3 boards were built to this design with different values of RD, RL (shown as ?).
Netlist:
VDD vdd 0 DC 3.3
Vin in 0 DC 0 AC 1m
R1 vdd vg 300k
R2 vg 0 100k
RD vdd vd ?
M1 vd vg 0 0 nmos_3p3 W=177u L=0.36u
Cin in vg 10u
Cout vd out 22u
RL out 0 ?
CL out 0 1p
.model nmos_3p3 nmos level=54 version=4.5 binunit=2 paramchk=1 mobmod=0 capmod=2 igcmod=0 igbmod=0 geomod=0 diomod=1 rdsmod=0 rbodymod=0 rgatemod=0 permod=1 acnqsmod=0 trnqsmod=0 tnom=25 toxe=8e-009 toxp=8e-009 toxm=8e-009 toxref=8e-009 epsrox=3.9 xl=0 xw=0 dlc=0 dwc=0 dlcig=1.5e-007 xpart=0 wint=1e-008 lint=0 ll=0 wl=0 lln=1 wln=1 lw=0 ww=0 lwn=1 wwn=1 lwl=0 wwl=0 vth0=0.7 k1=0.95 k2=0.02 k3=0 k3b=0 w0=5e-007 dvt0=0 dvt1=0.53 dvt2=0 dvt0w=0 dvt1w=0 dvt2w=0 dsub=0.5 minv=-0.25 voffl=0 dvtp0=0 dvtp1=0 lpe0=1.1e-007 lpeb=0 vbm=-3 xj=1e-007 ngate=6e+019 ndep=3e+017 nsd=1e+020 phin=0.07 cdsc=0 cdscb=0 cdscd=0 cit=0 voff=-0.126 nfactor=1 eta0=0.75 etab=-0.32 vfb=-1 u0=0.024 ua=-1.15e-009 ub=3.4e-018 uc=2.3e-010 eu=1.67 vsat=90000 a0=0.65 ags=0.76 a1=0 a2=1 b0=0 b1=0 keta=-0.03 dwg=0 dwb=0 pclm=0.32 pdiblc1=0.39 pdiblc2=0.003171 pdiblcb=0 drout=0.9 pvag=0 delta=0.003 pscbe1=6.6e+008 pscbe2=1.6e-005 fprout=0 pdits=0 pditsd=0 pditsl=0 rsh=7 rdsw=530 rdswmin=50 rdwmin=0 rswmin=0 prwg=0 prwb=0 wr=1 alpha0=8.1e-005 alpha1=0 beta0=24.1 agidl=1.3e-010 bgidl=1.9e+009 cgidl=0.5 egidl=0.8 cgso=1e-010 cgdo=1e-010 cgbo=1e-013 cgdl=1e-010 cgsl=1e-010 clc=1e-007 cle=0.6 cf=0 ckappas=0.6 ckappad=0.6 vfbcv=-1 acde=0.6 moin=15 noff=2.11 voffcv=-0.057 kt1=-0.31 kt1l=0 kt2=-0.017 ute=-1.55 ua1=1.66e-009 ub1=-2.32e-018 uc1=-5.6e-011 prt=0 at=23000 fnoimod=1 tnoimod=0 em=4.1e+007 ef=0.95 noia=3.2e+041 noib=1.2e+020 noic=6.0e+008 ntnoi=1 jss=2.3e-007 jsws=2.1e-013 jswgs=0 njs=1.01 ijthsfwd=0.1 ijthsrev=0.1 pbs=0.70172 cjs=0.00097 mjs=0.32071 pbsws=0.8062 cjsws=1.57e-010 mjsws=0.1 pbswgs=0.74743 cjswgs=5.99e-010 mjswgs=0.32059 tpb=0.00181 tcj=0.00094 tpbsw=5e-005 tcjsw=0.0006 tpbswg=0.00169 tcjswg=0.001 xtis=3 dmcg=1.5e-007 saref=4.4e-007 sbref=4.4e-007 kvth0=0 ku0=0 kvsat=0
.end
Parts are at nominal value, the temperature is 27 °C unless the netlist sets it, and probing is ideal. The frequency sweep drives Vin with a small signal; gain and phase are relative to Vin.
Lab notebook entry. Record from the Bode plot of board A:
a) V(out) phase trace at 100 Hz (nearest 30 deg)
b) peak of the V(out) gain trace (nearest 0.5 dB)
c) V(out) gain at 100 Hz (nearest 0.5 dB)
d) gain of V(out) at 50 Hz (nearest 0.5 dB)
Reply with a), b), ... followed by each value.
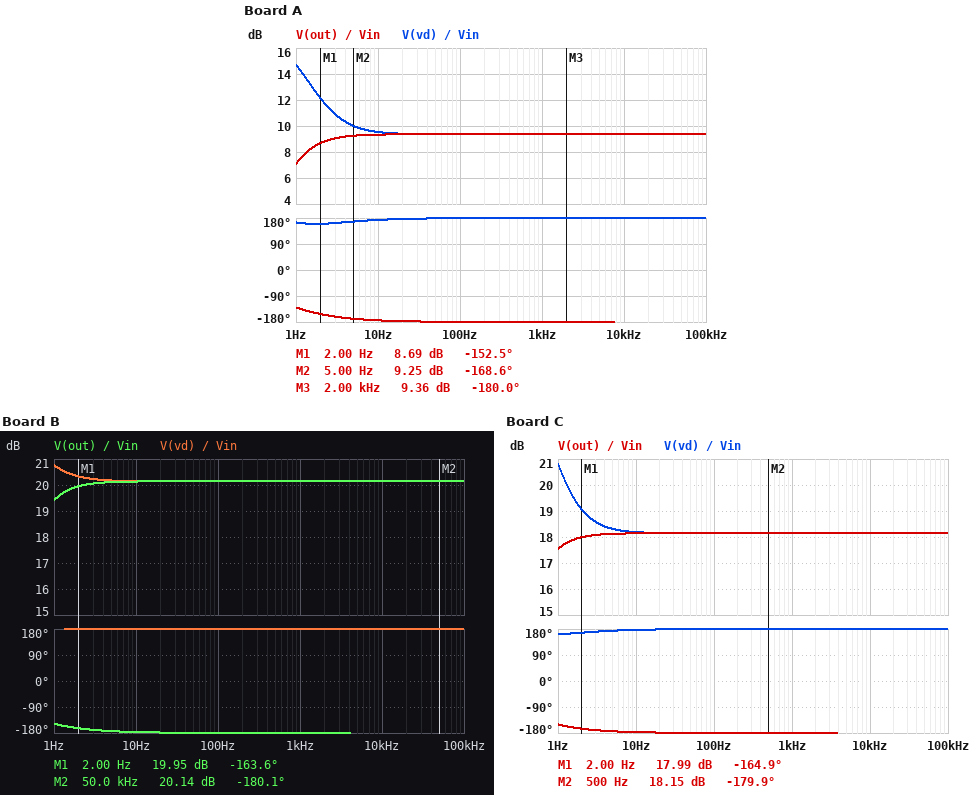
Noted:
a) -180 deg
b) 9.5 dB
c) 9.5 dB
d) 9.5 dB
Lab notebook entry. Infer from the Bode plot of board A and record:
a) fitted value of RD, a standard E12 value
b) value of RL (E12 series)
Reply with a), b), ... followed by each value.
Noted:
a) 39 kΩ
b) 3.3 kΩ
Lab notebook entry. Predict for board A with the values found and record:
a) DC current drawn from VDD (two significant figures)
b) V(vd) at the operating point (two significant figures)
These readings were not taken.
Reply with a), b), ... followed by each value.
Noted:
a) 91 µA
b) 83 mV
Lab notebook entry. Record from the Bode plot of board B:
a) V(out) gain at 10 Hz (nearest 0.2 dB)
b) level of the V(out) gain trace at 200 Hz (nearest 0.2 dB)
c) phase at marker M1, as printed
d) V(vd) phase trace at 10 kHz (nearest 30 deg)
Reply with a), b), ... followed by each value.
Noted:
a) 20.2 dB
b) 20.2 dB
c) -163.6 deg
d) 180 deg
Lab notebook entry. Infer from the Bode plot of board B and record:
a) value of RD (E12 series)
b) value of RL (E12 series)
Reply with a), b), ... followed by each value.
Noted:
a) 10 kΩ
b) 12 kΩ
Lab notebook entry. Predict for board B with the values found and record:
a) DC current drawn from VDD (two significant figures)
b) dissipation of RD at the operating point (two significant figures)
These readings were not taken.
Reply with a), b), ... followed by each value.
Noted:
a) 140 µA
b) 180 µW
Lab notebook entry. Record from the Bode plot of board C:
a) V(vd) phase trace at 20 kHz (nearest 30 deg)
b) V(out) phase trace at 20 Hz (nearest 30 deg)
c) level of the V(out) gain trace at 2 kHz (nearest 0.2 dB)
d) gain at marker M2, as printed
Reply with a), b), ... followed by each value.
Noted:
a) 180 deg
b) -180 deg
c) 18.2 dB
d) 18.15 dB
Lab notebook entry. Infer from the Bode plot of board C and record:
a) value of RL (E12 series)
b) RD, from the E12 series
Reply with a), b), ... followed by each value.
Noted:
a) 6.8 kΩ
b) 27 kΩ
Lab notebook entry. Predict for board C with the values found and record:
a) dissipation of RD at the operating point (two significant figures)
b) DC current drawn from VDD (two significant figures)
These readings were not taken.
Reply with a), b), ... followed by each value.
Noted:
a) 270 µW
b) 110 µA
